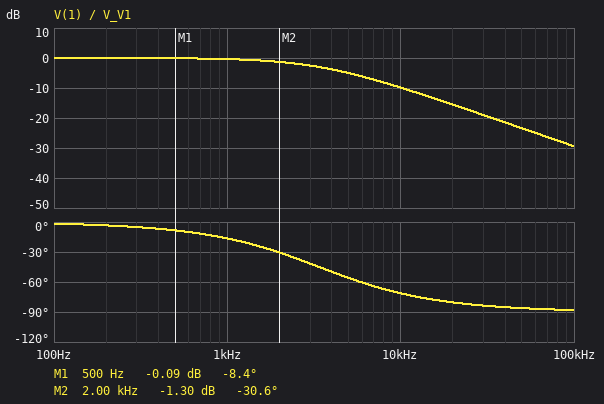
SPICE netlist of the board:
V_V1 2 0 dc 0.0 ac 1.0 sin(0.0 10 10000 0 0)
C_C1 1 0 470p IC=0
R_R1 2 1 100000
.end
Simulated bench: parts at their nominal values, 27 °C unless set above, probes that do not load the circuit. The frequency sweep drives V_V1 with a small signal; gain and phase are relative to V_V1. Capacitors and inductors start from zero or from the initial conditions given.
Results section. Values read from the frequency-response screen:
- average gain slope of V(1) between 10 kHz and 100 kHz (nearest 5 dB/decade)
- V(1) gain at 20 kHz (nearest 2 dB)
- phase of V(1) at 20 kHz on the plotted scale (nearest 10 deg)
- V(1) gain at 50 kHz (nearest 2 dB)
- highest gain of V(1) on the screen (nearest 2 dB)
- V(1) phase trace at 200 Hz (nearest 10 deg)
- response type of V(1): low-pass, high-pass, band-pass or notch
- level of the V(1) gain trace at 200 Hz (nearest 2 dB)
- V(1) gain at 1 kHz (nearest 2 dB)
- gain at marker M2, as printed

-20 dB/decade
-16 dB
-80 deg
-24 dB
0 dB
0 deg
low-pass
0 dB
0 dB
-1.30 dB
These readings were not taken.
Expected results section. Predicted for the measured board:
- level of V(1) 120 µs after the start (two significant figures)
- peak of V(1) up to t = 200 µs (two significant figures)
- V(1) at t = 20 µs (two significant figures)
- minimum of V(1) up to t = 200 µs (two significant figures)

280 mV
4.4 V
2.0 V
-3.2 V
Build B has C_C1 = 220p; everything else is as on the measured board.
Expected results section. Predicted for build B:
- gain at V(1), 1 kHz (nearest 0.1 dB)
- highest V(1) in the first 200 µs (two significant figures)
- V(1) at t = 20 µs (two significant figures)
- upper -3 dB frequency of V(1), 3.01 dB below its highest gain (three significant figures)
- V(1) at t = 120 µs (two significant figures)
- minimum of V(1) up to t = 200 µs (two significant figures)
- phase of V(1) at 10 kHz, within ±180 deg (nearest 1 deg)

-0.1 dB
6.7 V
3.7 V
7.23 kHz
1.8 V
-5.9 V
-54 deg
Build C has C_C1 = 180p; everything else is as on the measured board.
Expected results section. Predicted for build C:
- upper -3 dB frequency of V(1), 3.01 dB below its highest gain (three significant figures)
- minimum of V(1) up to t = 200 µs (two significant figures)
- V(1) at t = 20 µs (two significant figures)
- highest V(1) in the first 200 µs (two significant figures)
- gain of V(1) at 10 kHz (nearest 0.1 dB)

8.84 kHz
-6.6 V
4.3 V
7.2 V
-3.6 dB
